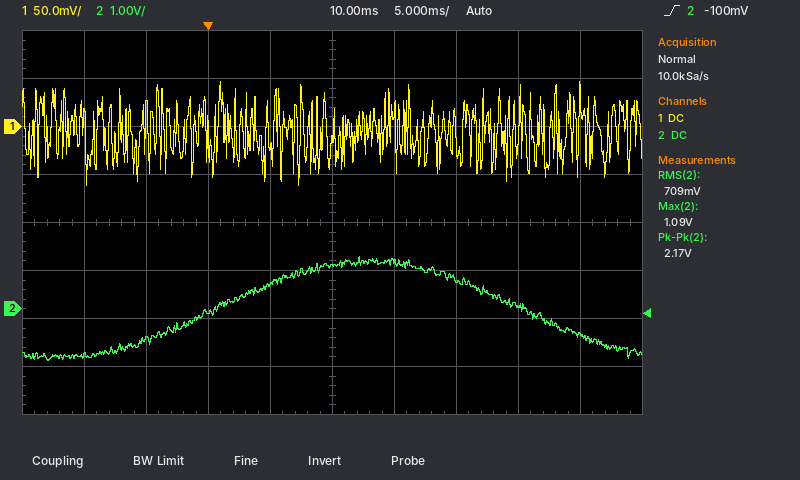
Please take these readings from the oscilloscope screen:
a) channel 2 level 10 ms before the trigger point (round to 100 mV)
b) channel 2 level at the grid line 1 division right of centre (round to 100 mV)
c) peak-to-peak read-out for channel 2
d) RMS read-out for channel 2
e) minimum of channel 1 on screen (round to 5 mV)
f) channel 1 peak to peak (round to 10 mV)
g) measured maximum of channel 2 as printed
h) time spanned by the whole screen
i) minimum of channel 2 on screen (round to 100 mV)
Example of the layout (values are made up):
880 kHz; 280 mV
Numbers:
-1.0 V; 1.0 V; 2.17 V; 709 mV; -60 mV; 110 mV; 1.09 V; 50 ms; -1.1 V
